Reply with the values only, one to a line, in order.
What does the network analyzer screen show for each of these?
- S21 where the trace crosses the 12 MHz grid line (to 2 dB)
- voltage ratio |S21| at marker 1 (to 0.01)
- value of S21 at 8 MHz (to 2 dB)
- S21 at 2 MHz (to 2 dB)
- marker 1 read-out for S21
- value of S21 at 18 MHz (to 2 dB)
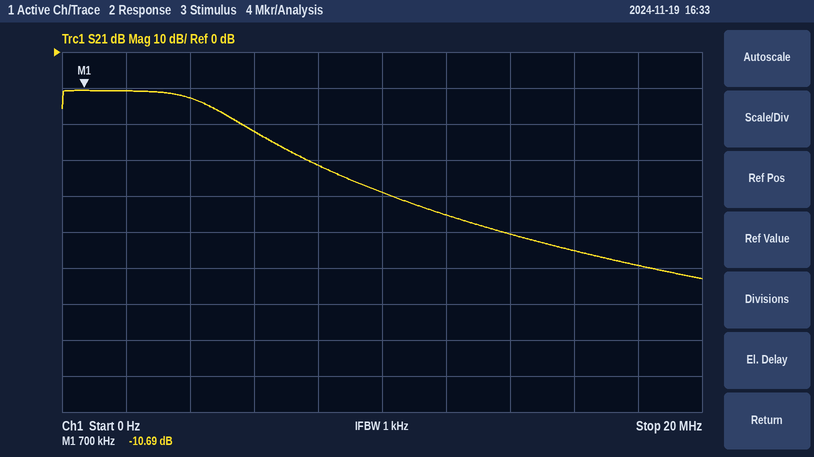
-46 dB
0.29
-32 dB
-10 dB
-10.69 dB
-60 dB
